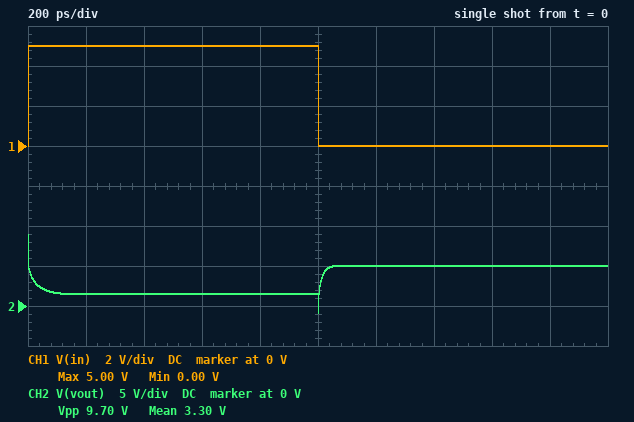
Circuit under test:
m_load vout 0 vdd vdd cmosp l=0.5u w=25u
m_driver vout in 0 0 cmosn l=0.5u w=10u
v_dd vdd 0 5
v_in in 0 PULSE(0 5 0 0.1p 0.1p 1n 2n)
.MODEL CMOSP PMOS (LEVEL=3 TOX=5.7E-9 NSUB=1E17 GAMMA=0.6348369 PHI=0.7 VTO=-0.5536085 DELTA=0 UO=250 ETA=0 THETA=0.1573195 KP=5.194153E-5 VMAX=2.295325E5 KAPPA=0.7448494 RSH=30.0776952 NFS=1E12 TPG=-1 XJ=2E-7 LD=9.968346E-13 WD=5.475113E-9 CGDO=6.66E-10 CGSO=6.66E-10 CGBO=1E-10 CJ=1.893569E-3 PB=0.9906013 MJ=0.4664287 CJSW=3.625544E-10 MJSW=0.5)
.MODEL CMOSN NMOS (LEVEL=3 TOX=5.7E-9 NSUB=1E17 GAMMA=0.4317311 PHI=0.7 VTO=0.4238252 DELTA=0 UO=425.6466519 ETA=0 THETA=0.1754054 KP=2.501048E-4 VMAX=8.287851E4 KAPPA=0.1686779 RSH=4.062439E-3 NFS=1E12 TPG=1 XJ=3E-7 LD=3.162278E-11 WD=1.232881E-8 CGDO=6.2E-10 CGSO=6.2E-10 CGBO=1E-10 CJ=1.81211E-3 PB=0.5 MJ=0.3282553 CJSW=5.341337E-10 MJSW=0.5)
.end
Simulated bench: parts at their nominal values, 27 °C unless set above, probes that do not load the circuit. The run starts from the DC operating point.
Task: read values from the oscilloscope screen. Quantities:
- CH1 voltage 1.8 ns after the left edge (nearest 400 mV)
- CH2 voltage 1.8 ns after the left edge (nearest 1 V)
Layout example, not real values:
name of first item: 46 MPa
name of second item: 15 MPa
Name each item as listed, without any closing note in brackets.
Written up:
CH1 voltage 1.8 ns after the left edge: 0 V
CH2 voltage 1.8 ns after the left edge: 5 V
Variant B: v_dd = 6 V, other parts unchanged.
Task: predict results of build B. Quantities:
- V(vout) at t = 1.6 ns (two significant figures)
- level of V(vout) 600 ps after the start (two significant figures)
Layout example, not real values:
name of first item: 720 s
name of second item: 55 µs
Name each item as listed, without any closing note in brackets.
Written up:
V(vout) at t = 1.6 ns: 6.0 V
level of V(vout) 600 ps after the start: 3.4 V
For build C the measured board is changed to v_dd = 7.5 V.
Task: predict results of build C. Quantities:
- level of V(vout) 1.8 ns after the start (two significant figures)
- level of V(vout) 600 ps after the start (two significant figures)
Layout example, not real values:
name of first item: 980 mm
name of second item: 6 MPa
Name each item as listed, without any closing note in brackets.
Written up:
level of V(vout) 1.8 ns after the start: 7.5 V
level of V(vout) 600 ps after the start: 5.3 V
